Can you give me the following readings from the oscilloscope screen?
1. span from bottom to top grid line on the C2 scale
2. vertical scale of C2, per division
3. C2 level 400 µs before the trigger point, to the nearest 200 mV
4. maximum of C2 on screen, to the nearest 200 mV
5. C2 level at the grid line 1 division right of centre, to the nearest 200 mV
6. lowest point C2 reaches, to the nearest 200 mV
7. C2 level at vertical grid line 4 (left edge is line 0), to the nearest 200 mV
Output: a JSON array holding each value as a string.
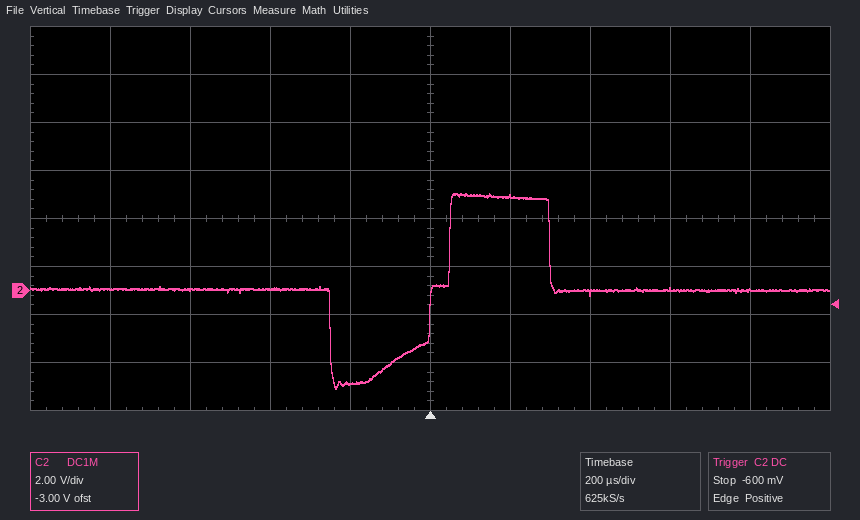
["16 V", "2 V", "0.0 V", "4.0 V", "4.0 V", "-4.0 V", "-3.8 V"]
